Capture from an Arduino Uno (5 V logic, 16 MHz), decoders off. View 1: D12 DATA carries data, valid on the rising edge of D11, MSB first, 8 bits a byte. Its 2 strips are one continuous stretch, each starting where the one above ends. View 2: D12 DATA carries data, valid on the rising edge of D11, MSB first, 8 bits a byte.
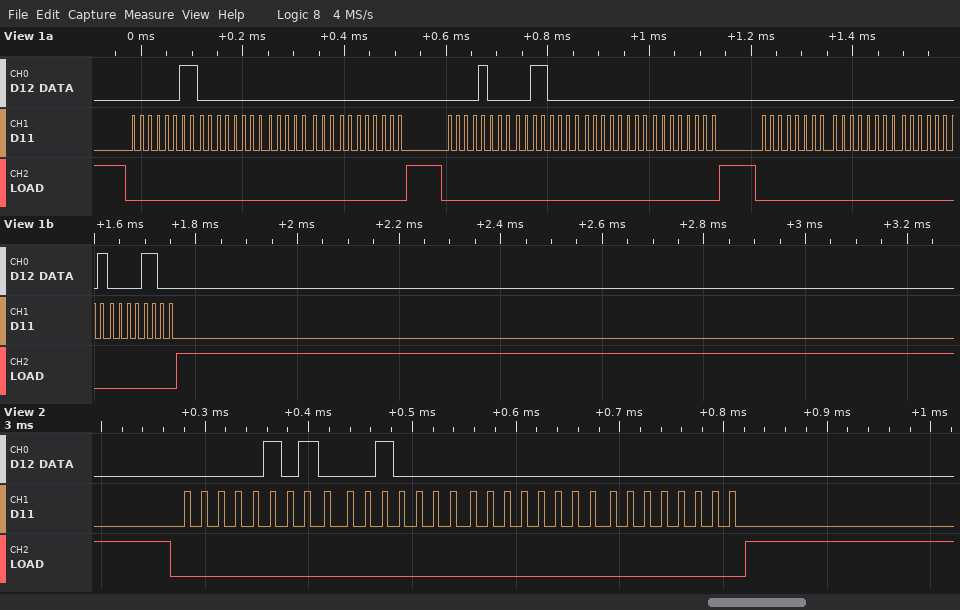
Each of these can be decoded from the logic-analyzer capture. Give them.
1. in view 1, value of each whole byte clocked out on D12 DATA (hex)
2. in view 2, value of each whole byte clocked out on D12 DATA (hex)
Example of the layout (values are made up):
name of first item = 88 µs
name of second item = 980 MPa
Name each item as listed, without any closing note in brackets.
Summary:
in view 1, value of each whole byte clocked out on D12 DATA = 03 00 00 00 08 30 00 00 00 00 01 0C
in view 2, value of each whole byte clocked out on D12 DATA = 05 10 00 00
